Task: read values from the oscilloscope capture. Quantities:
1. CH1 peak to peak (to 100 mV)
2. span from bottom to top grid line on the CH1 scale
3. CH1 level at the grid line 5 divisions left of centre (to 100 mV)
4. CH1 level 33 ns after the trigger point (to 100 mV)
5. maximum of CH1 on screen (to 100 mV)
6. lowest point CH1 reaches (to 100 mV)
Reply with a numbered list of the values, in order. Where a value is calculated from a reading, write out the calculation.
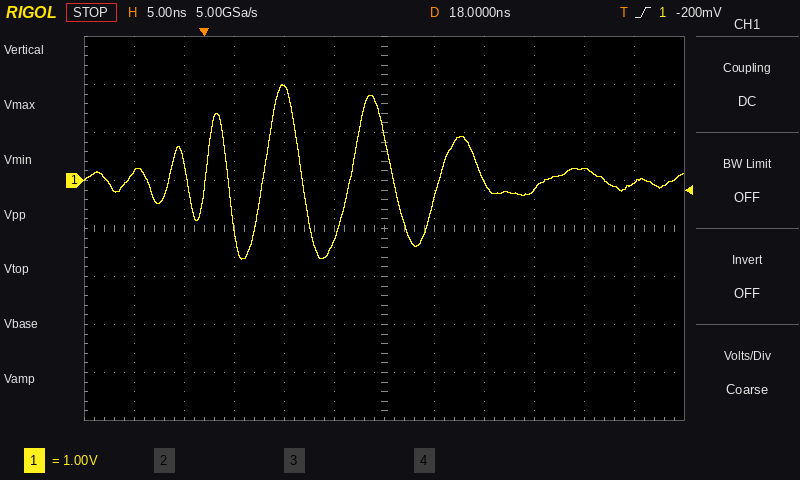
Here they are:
1. 2.0 V − (-1.6 V) = 3.6 V
2. 8 V
3. 200 mV
4. -200 mV
5. 2.0 V
6. -1.6 V
